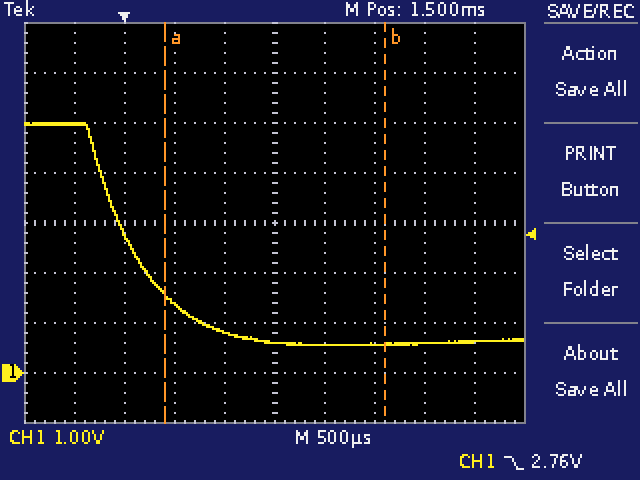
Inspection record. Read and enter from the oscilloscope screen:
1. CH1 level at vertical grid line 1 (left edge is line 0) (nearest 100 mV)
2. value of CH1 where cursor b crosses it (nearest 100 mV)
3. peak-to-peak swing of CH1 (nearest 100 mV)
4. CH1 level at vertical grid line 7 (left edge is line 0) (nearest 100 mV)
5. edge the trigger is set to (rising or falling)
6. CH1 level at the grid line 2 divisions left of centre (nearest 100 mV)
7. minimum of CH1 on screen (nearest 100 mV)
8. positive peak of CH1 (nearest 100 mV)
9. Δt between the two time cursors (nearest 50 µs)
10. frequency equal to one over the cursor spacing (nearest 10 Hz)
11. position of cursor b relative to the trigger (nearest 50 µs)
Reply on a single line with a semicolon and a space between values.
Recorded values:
5.0 V; 600 mV; 4.4 V; 600 mV; falling; 1.4 V; 600 mV; 5.0 V; 2.20 ms; 450 Hz; +2.60 ms
